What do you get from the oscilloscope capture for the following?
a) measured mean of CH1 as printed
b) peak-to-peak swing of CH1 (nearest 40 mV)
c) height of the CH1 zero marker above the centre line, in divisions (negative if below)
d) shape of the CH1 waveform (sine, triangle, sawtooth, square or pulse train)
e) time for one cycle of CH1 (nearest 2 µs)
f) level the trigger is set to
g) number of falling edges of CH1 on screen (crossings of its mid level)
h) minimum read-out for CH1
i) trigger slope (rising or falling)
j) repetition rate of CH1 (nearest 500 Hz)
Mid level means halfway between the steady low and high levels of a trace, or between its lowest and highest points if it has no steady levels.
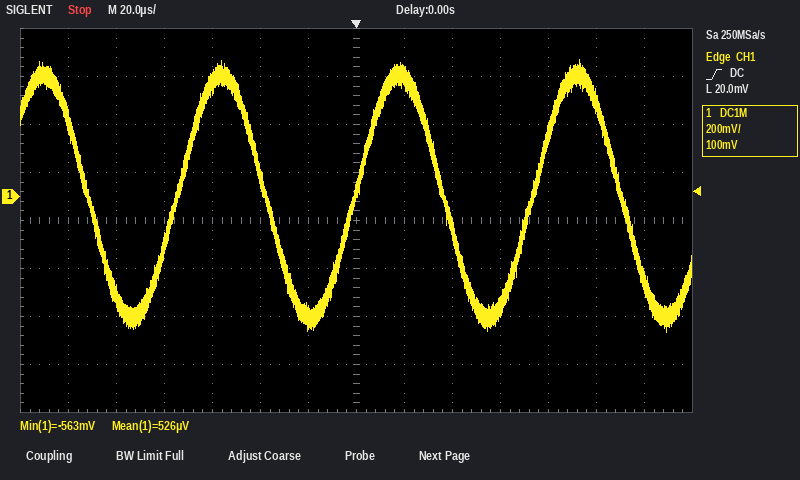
526 µV
1.12 V
+0.5 div
sine
74 µs
20.0 mV
4
-563 mV
rising
13.5 kHz
